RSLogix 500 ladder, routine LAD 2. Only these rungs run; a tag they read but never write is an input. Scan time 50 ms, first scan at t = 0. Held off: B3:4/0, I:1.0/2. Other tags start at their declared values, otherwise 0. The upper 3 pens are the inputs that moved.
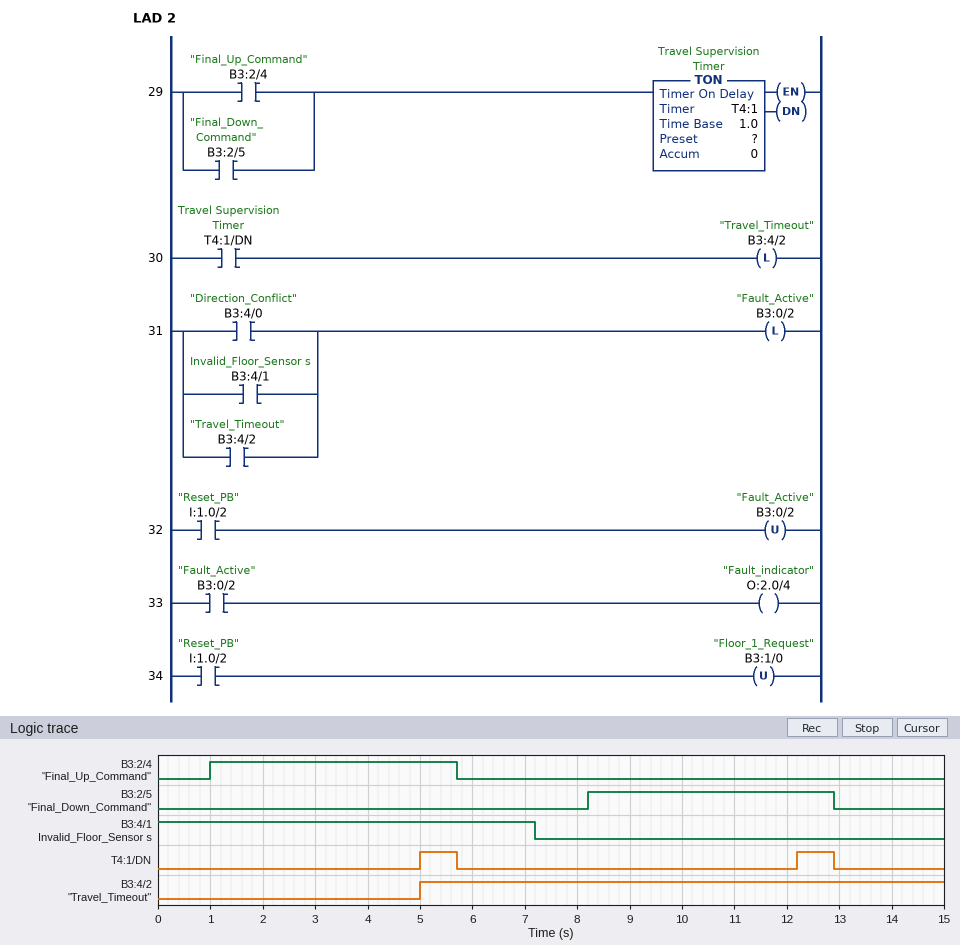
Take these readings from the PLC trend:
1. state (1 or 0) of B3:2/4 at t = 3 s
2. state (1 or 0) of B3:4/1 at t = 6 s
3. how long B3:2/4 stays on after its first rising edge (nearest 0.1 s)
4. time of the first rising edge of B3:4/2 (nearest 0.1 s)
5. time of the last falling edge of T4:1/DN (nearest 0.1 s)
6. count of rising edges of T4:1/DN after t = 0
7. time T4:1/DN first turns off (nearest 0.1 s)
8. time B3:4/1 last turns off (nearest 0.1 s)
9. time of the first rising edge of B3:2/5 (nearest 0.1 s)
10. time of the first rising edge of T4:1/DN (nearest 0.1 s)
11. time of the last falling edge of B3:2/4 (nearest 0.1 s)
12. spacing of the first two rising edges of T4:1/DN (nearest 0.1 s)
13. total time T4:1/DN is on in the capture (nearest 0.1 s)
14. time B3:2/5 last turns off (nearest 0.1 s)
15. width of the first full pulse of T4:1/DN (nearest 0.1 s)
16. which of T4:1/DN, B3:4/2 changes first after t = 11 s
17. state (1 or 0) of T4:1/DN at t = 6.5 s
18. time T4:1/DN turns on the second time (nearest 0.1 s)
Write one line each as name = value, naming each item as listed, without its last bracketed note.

state (1 or 0) of B3:2/4 at t = 3 s = 1
state (1 or 0) of B3:4/1 at t = 6 s = 1
how long B3:2/4 stays on after its first rising edge = 4.7 s
time of the first rising edge of B3:4/2 = 5.0 s
time of the last falling edge of T4:1/DN = 12.9 s
count of rising edges of T4:1/DN after t = 0 = 2
time T4:1/DN first turns off = 5.7 s
time B3:4/1 last turns off = 7.2 s
time of the first rising edge of B3:2/5 = 8.2 s
time of the first rising edge of T4:1/DN = 5.0 s
time of the last falling edge of B3:2/4 = 5.7 s
spacing of the first two rising edges of T4:1/DN = 7.2 s
total time T4:1/DN is on in the capture = 1.4 s
time B3:2/5 last turns off = 12.9 s
width of the first full pulse of T4:1/DN = 0.7 s
which of T4:1/DN, B3:4/2 changes first after t = 11 s = T4:1/DN
state (1 or 0) of T4:1/DN at t = 6.5 s = 0
time T4:1/DN turns on the second time = 12.2 s
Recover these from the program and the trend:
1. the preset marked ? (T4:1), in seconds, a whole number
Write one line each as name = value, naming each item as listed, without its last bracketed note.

the preset marked ? (T4:1), in seconds, a whole number = 4 s
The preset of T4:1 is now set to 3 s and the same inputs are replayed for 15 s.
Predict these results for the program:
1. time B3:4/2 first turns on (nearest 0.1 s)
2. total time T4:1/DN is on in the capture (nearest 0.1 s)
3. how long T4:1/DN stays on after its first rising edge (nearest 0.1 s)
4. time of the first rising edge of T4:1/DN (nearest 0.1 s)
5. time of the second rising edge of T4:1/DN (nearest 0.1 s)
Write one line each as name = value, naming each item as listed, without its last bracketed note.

time B3:4/2 first turns on = 4.0 s
total time T4:1/DN is on in the capture = 3.4 s
how long T4:1/DN stays on after its first rising edge = 1.7 s
time of the first rising edge of T4:1/DN = 4.0 s
time of the second rising edge of T4:1/DN = 11.2 s
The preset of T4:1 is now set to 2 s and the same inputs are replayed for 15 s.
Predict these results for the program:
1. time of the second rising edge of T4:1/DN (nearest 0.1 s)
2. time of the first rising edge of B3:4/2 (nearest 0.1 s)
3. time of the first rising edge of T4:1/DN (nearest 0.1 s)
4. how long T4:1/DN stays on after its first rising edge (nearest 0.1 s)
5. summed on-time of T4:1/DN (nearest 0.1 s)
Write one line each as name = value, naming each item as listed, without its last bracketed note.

time of the second rising edge of T4:1/DN = 10.2 s
time of the first rising edge of B3:4/2 = 3.0 s
time of the first rising edge of T4:1/DN = 3.0 s
how long T4:1/DN stays on after its first rising edge = 2.7 s
summed on-time of T4:1/DN = 5.4 s
